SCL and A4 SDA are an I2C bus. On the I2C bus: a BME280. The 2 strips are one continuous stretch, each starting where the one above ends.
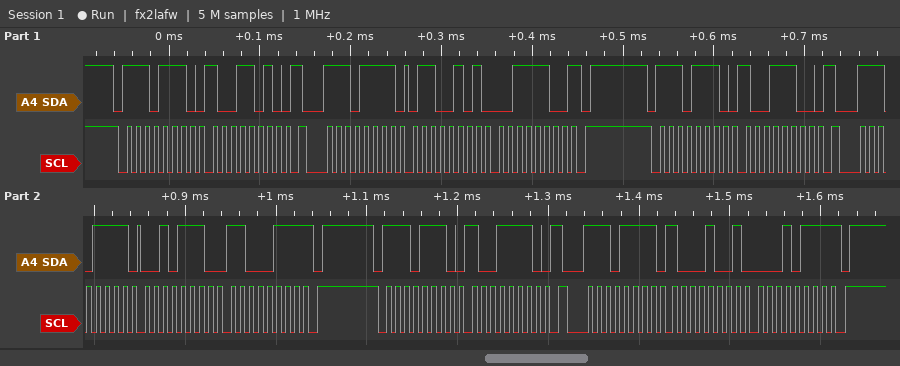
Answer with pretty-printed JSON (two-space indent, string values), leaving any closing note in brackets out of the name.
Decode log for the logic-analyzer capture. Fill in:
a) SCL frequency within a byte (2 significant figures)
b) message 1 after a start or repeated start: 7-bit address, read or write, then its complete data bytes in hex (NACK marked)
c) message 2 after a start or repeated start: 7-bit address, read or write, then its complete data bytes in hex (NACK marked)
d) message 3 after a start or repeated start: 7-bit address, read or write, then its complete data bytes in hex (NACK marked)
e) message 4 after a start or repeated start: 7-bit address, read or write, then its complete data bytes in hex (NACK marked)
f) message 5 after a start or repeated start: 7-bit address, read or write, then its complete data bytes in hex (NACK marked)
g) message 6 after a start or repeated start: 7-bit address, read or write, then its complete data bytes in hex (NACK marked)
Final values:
{
  "SCL frequency within a byte": "100 kHz",
  "message 1 after a start or repeated start: 7-bit address, read or write, then its complete data bytes in hex": "0x77 write: 9A",
  "message 2 after a start or repeated start: 7-bit address, read or write, then its complete data bytes in hex": "0x77 read: 65 3C NACK",
  "message 3 after a start or repeated start: 7-bit address, read or write, then its complete data bytes in hex": "0x77 write: 9C",
  "message 4 after a start or repeated start: 7-bit address, read or write, then its complete data bytes in hex": "0x77 read: 2E C7 NACK",
  "message 5 after a start or repeated start: 7-bit address, read or write, then its complete data bytes in hex": "0x77 write: 9E",
  "message 6 after a start or repeated start: 7-bit address, read or write, then its complete data bytes in hex": "0x77 read: 89 17 NACK"
}
